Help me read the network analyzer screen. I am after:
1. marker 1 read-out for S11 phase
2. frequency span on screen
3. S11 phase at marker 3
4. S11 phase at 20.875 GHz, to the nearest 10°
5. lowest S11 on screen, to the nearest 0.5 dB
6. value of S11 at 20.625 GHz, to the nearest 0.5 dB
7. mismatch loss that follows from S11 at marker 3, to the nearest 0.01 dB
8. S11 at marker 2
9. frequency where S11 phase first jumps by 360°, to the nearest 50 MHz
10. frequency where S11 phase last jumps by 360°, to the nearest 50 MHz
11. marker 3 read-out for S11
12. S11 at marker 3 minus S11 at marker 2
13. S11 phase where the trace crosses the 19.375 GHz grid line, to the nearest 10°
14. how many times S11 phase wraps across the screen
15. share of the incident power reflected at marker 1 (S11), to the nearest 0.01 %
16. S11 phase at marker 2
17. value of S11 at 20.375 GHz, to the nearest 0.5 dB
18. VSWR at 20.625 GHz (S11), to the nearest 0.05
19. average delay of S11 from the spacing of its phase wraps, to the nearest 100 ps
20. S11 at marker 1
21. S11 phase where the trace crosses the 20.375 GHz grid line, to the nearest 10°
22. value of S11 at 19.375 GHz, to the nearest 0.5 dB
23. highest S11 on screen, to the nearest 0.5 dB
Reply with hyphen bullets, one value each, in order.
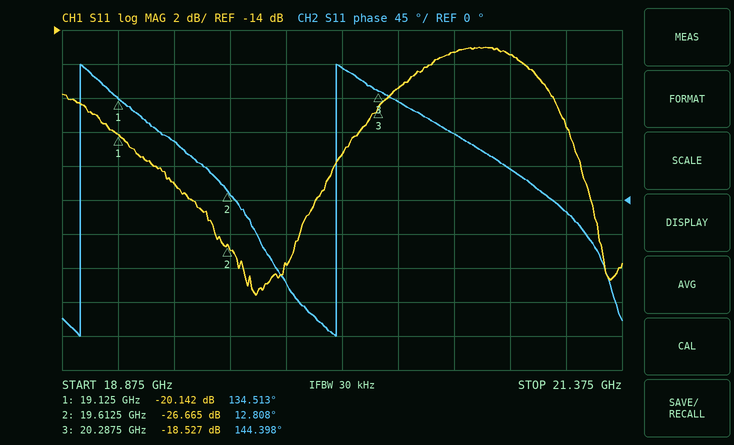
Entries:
- 134.513°
- 2.5 GHz
- 144.398°
- 40°
- -29.5 dB
- -15.5 dB
- 0.06 dB
- -26.665 dB
- 18.95 GHz
- 20.10 GHz
- -18.527 dB
- 8.138 dB
- 80°
- 2
- 0.97 %
- 12.808°
- -17.5 dB
- 1.40
- 900 ps
- -20.142 dB
- 130°
- -23.0 dB
- -15.0 dB
